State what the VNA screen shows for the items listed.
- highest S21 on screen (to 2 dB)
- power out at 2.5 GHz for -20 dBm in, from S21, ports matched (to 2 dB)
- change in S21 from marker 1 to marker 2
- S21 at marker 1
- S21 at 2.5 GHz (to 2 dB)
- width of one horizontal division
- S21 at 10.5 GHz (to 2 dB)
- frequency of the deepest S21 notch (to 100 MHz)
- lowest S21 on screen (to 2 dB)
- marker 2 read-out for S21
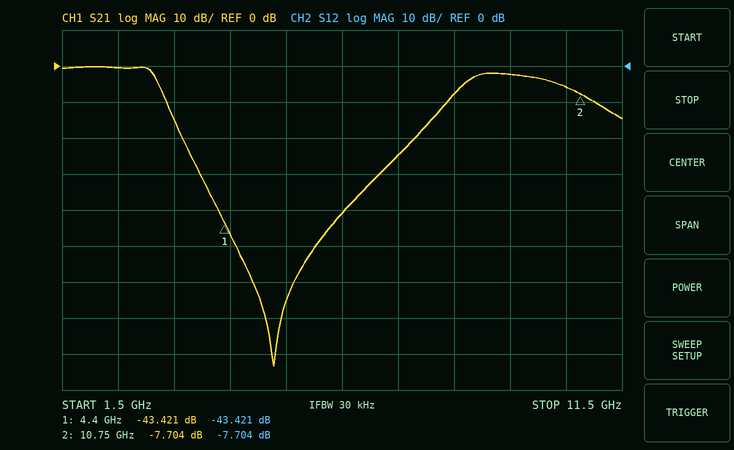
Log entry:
0 dB
-20 dBm
35.717 dB
-43.421 dB
0 dB
1 GHz
-6 dB
5.3 GHz
-84 dB
-7.704 dB
